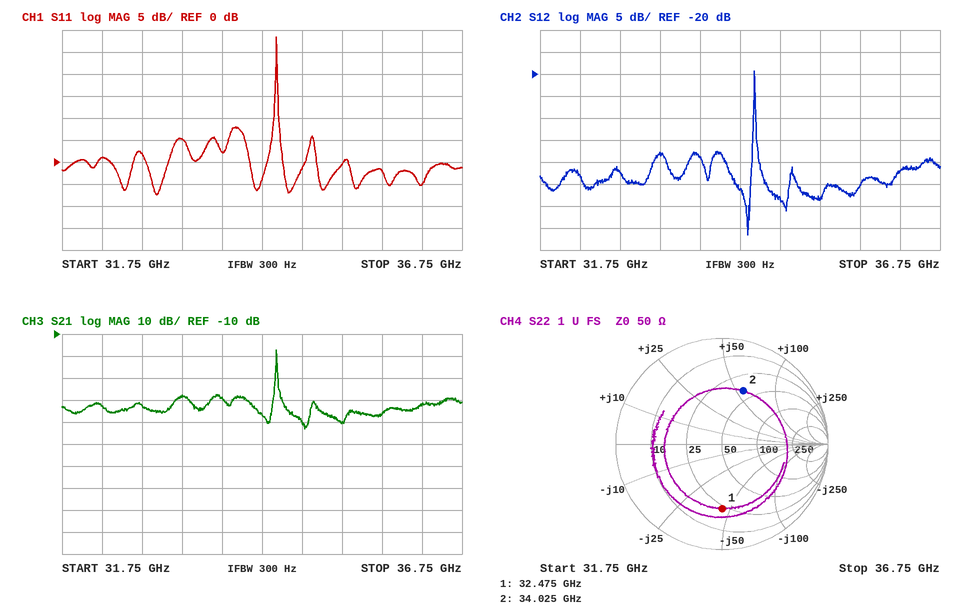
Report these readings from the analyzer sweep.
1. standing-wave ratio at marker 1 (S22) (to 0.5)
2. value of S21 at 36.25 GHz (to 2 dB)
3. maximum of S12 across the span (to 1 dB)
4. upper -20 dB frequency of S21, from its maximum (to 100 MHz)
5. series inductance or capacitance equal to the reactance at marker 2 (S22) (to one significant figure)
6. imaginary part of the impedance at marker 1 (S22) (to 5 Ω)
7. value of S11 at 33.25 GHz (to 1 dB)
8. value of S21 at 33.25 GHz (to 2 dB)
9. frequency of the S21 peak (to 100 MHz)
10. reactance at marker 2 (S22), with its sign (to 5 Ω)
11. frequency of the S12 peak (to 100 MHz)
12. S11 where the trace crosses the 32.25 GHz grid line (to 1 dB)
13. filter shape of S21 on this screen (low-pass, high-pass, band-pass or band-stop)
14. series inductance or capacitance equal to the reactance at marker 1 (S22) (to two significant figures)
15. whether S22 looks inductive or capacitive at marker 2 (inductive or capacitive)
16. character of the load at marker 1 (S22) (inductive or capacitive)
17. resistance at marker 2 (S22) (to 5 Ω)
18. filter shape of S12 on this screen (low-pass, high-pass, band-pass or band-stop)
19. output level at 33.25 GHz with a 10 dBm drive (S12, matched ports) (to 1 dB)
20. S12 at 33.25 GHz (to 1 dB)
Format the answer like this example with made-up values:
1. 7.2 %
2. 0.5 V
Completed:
1. 4.0
2. -42 dB
3. -19 dB
4. 34.5 GHz
5. 300 pH
6. -45 Ω
7. 5 dB
8. -38 dB
9. 34.4 GHz
10. +55 Ω
11. 34.4 GHz
12. 1 dB
13. band-pass
14. 110 fF
15. inductive
16. capacitive
17. 40 Ω
18. band-pass
19. -28 dBm
20. -38 dB
